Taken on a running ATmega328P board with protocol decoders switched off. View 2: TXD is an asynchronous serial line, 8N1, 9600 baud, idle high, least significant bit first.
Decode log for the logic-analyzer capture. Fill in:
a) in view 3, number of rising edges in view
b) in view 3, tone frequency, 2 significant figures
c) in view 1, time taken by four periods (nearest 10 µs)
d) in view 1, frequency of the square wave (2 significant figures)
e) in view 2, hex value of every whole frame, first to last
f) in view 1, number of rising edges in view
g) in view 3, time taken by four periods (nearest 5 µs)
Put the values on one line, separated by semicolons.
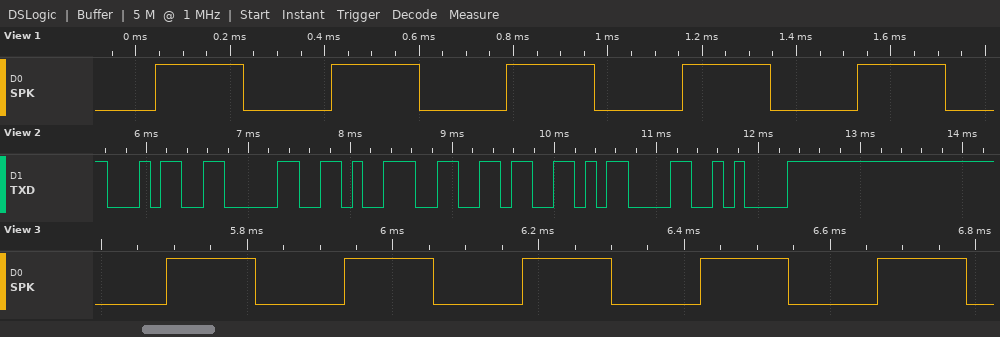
5; 4.1 kHz; 1490 µs; 2.7 kHz; 34 30 39 36 0D 0A; 5; 975 µs
